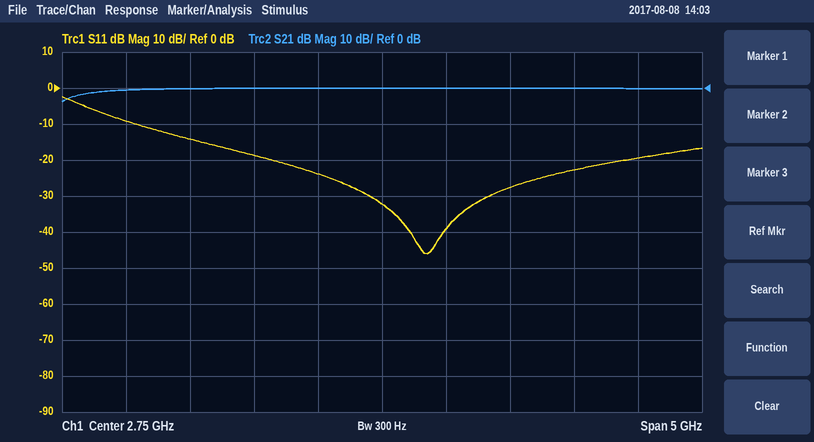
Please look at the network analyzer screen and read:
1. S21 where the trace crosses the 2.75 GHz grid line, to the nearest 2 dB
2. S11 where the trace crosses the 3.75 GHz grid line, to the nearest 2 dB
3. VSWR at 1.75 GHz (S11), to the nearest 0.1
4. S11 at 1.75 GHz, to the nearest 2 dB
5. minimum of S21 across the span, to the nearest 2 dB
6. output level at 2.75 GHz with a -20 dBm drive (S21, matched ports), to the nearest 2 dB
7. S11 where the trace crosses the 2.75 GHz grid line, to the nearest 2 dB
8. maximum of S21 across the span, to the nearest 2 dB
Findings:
0 dB
-28 dB
1.3
-18 dB
-4 dB
-20 dBm
-32 dB
0 dB
